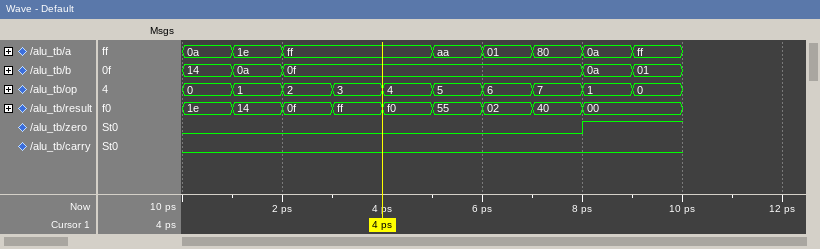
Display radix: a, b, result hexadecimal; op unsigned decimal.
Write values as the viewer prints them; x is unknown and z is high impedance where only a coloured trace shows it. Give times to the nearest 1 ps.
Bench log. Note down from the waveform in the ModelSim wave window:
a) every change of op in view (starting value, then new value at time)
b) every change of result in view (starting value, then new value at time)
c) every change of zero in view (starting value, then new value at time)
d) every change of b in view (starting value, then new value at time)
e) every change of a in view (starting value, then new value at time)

0, 1 at 1 ps, 2 at 2 ps, 3 at 3 ps, 4 at 4 ps, 5 at 5 ps, 6 at 6 ps, 7 at 7 ps, 1 at 8 ps, 0 at 9 ps
1e, 14 at 1 ps, 0f at 2 ps, ff at 3 ps, f0 at 4 ps, 55 at 5 ps, 02 at 6 ps, 40 at 7 ps, 00 at 8 ps
0, 1 at 8 ps
14, 0a at 1 ps, 0f at 2 ps, 0a at 8 ps, 01 at 9 ps
0a, 1e at 1 ps, ff at 2 ps, aa at 5 ps, 01 at 6 ps, 80 at 7 ps, 0a at 8 ps, ff at 9 ps
